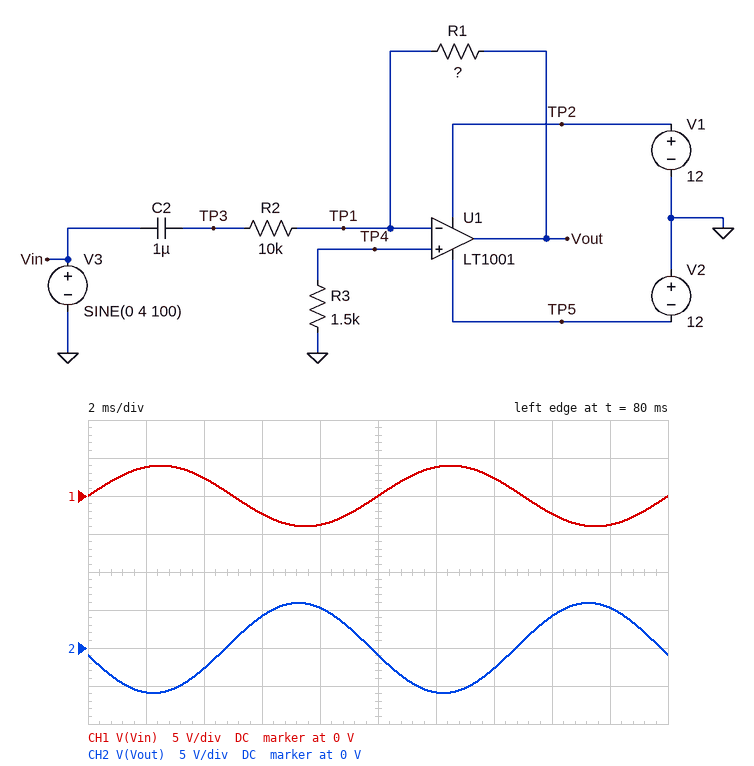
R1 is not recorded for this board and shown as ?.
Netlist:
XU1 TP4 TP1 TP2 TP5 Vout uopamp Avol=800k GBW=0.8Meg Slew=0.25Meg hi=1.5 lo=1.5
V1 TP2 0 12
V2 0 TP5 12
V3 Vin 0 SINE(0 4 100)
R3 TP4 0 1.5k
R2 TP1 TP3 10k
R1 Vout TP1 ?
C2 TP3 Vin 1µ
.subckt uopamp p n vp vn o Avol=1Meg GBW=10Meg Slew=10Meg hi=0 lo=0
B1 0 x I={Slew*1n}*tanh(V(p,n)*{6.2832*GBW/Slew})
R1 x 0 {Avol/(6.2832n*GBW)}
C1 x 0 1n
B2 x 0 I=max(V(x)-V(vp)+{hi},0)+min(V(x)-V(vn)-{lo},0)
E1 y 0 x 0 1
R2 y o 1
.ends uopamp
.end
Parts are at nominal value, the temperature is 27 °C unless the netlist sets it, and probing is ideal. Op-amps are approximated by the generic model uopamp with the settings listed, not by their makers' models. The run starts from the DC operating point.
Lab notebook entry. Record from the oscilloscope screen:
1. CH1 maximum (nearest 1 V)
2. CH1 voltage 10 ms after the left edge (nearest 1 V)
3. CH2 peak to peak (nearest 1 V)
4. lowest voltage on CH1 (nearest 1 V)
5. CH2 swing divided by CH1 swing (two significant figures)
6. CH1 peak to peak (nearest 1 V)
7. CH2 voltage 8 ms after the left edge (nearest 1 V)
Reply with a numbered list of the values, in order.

1. 4 V
2. 0 V
3. 12 V
4. -4 V
5. 1.5
6. 8 V
7. 5 V
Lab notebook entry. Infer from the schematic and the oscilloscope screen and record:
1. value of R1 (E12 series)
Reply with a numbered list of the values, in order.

1. 15 kΩ
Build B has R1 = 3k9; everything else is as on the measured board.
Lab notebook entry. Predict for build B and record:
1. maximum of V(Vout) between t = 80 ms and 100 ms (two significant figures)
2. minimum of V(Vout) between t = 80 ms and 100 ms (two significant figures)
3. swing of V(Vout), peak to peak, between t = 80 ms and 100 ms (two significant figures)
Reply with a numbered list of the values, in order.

1. 1.5 V
2. -1.5 V
3. 3.1 V
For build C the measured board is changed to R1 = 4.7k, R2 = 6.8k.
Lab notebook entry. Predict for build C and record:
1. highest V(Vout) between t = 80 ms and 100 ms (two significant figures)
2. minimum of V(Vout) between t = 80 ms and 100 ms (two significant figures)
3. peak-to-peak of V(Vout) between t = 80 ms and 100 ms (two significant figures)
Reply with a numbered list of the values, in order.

1. 2.7 V
2. -2.7 V
3. 5.4 V
